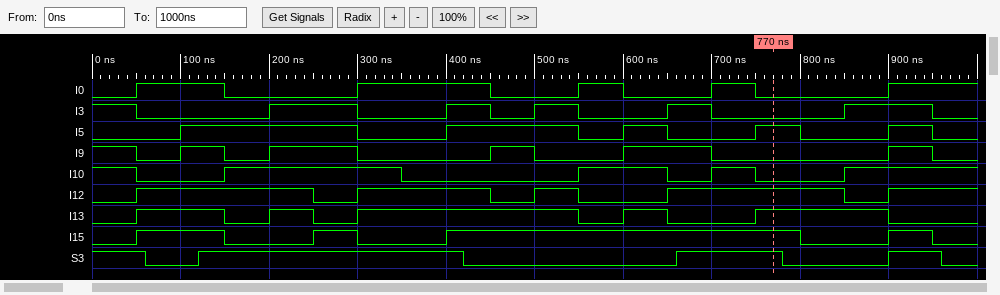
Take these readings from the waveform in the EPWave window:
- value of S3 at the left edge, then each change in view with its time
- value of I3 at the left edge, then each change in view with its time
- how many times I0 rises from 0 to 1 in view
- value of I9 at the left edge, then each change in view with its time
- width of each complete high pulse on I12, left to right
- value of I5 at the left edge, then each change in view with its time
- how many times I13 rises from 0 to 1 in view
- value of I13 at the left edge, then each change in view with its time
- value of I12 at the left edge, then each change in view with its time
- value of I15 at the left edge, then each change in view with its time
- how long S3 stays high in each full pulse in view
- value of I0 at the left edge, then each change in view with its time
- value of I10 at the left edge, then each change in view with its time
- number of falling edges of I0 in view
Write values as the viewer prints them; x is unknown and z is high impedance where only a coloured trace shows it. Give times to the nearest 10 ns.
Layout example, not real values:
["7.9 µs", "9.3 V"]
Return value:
["1, 0 at 60 ns, 1 at 120 ns, 0 at 420 ns, 1 at 660 ns, 0 at 780 ns, 1 at 900 ns, 0 at 960 ns", "1, 0 at 50 ns, 1 at 200 ns, 0 at 300 ns, 1 at 400 ns, 0 at 450 ns, 1 at 500 ns, 0 at 550 ns, 1 at 650 ns, 0 at 700 ns, 1 at 850 ns, 0 at 950 ns", "5", "1, 0 at 50 ns, 1 at 100 ns, 0 at 150 ns, 1 at 200 ns, 0 at 300 ns, 1 at 450 ns, 0 at 500 ns, 1 at 600 ns, 0 at 700 ns, 1 at 900 ns, 0 at 950 ns", "200 ns, 150 ns, 50 ns, 200 ns", "0, 1 at 100 ns, 0 at 300 ns, 1 at 400 ns, 0 at 550 ns, 1 at 600 ns, 0 at 650 ns, 1 at 750 ns, 0 at 800 ns, 1 at 900 ns, 0 at 950 ns", "5", "0, 1 at 50 ns, 0 at 150 ns, 1 at 200 ns, 0 at 250 ns, 1 at 300 ns, 0 at 550 ns, 1 at 600 ns, 0 at 650 ns, 1 at 750 ns, 0 at 900 ns", "0, 1 at 50 ns, 0 at 250 ns, 1 at 300 ns, 0 at 450 ns, 1 at 500 ns, 0 at 550 ns, 1 at 650 ns, 0 at 850 ns, 1 at 900 ns", "0, 1 at 50 ns, 0 at 150 ns, 1 at 250 ns, 0 at 300 ns, 1 at 400 ns, 0 at 800 ns, 1 at 900 ns, 0 at 950 ns", "300 ns, 120 ns, 60 ns", "0, 1 at 50 ns, 0 at 150 ns, 1 at 300 ns, 0 at 450 ns, 1 at 550 ns, 0 at 600 ns, 1 at 700 ns, 0 at 750 ns, 1 at 900 ns", "1, 0 at 50 ns, 1 at 150 ns, 0 at 350 ns, 1 at 550 ns, 0 at 650 ns, 1 at 700 ns, 0 at 750 ns, 1 at 850 ns", "4"]
